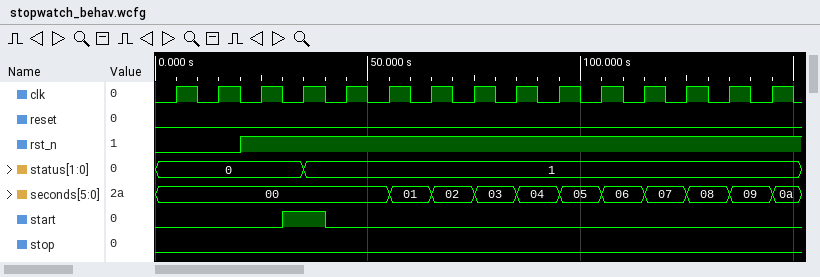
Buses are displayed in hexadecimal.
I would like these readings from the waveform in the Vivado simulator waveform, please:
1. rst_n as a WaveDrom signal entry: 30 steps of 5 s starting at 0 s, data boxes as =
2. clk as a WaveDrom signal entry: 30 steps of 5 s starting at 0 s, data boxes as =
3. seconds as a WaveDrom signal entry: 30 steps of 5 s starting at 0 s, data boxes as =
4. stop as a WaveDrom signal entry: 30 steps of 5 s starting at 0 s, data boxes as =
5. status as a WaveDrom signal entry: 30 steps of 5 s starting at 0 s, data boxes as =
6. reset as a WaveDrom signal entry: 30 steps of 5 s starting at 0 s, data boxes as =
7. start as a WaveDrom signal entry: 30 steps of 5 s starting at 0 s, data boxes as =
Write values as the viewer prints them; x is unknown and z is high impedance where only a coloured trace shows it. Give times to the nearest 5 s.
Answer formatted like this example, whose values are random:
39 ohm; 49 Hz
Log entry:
{name: 'rst_n', wave: '0...1.........................'}; {name: 'clk', wave: '010101010101010101010101010101'}; {name: 'seconds', wave: '=..........=.=.=.=.=.=.=.=.=.=', data: '00 01 02 03 04 05 06 07 08 09 0a'}; {name: 'stop', wave: '0.............................'}; {name: 'status', wave: '=......=......................', data: '0 1'}; {name: 'reset', wave: '0.............................'}; {name: 'start', wave: '0.....1.0.....................'}
